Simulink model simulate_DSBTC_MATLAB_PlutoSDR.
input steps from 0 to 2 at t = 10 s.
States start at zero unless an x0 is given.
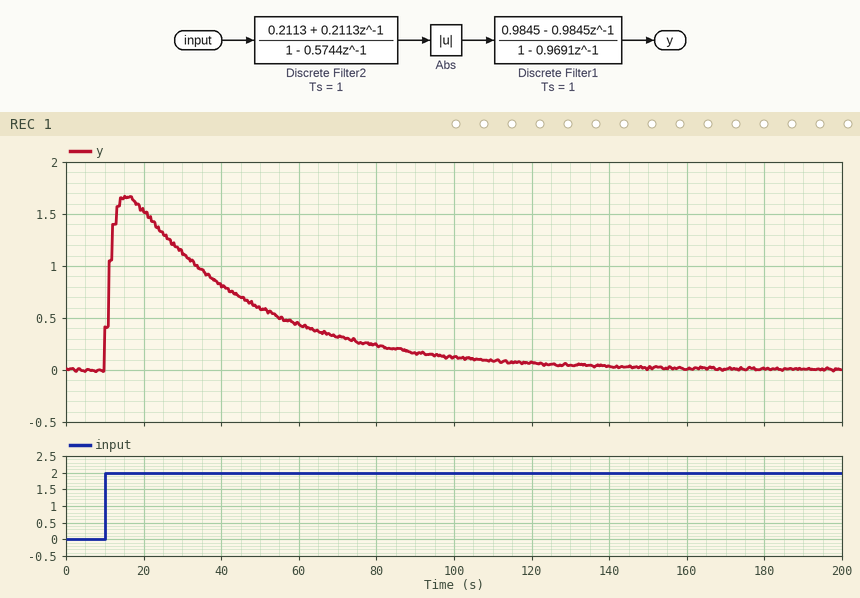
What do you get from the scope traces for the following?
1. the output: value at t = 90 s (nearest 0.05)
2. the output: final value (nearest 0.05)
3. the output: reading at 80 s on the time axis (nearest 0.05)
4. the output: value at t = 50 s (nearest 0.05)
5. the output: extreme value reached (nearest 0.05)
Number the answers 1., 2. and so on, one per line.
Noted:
1. 0.15
2. 0.00
3. 0.25
4. 0.60
5. 1.65
